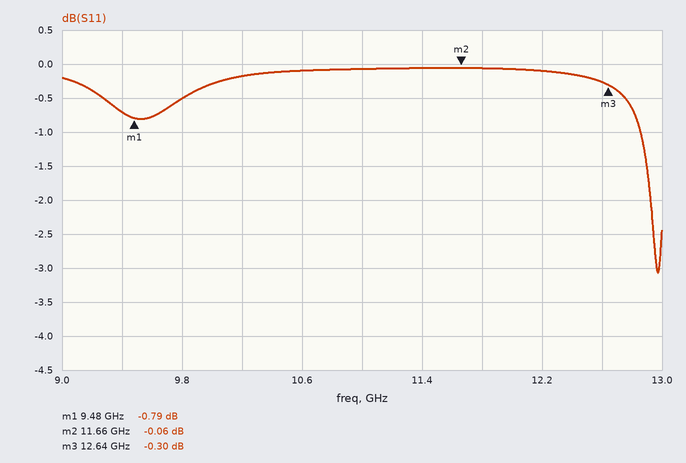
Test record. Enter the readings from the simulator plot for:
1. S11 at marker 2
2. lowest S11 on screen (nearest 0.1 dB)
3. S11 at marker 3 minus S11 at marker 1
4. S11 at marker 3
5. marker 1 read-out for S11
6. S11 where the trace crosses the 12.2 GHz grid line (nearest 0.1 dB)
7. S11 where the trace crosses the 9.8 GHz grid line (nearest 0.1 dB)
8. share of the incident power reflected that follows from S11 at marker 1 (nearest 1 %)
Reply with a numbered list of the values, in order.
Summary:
1. -0.06 dB
2. -3.1 dB
3. 0.49 dB
4. -0.30 dB
5. -0.79 dB
6. -0.1 dB
7. -0.5 dB
8. 83 %
